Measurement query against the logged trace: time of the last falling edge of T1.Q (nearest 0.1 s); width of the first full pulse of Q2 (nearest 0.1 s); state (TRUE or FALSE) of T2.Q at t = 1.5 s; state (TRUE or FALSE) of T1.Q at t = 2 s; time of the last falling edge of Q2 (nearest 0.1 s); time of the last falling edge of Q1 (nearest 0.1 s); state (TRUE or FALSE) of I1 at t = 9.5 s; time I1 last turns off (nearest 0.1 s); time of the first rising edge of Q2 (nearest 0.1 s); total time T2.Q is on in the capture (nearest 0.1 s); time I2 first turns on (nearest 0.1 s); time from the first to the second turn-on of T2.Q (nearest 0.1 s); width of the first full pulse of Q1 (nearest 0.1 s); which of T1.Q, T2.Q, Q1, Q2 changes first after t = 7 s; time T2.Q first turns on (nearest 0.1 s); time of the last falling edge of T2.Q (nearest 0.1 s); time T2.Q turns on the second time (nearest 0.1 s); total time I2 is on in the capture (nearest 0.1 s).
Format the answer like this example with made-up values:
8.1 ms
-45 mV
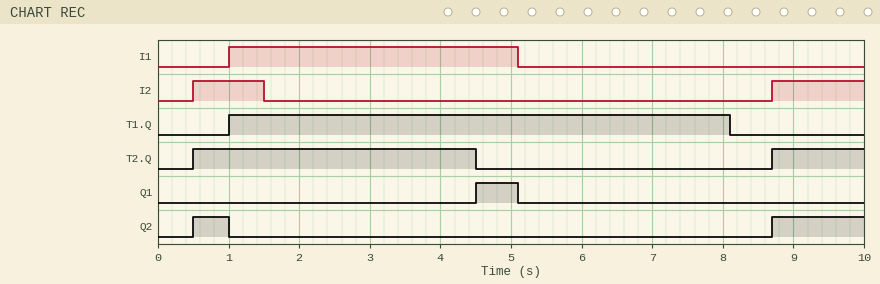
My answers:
8.1 s
0.5 s
TRUE
TRUE
1.0 s
5.1 s
FALSE
5.1 s
0.5 s
5.3 s
0.5 s
8.2 s
0.6 s
T1.Q
0.5 s
4.5 s
8.7 s
2.3 s
